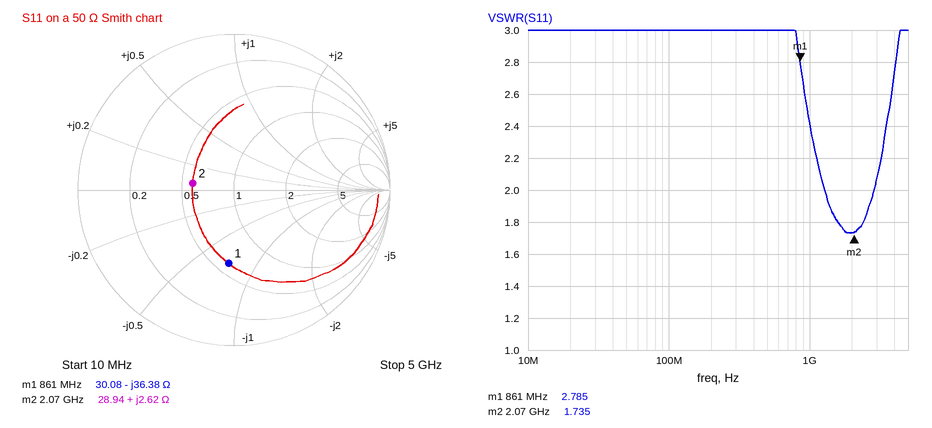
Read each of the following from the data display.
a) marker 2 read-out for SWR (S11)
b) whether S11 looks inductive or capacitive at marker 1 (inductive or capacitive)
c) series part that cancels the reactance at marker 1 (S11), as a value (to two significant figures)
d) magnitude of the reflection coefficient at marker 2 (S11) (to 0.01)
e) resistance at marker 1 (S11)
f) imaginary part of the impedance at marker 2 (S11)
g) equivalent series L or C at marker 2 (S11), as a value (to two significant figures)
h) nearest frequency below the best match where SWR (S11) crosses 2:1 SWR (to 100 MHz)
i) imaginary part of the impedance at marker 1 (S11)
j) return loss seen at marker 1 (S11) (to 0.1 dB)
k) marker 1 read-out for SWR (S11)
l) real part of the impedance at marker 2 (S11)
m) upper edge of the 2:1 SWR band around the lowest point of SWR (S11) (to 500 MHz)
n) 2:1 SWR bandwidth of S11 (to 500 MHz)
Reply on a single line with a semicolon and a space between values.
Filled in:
1.735; capacitive; 6.7 nH; 0.27; 30.08 Ω; +2.62 Ω; 200 pH; 1.3 GHz; -36.38 Ω; 6.5 dB; 2.785; 28.94 Ω; 3.0 GHz; 1.5 GHz
